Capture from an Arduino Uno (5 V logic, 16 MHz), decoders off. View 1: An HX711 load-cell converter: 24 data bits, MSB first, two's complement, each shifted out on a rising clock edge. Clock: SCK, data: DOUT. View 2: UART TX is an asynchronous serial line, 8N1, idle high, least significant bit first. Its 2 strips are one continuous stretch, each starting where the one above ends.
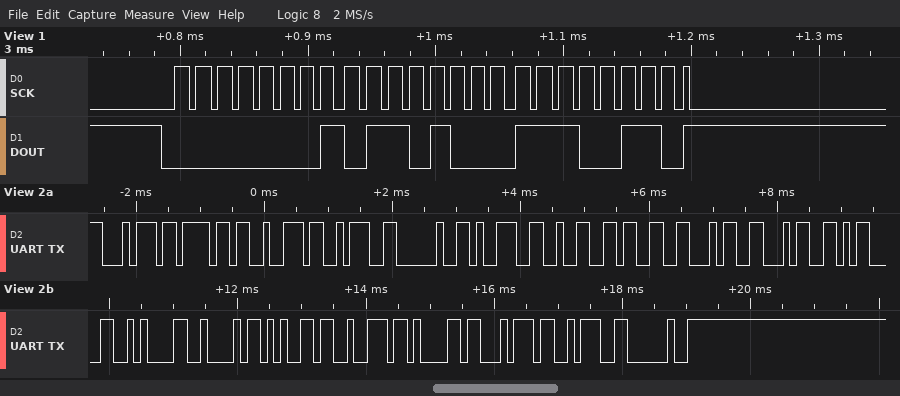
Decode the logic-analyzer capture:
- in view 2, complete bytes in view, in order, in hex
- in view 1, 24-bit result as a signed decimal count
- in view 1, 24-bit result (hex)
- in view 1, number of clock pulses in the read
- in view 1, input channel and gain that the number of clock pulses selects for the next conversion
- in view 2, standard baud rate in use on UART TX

74 6F 72 3A 20 39 32 33 34 34 0D 0A 42 65 72 61 74 3A 20
92390
0x0168E6
25
channel A, gain 128
9600 baud
